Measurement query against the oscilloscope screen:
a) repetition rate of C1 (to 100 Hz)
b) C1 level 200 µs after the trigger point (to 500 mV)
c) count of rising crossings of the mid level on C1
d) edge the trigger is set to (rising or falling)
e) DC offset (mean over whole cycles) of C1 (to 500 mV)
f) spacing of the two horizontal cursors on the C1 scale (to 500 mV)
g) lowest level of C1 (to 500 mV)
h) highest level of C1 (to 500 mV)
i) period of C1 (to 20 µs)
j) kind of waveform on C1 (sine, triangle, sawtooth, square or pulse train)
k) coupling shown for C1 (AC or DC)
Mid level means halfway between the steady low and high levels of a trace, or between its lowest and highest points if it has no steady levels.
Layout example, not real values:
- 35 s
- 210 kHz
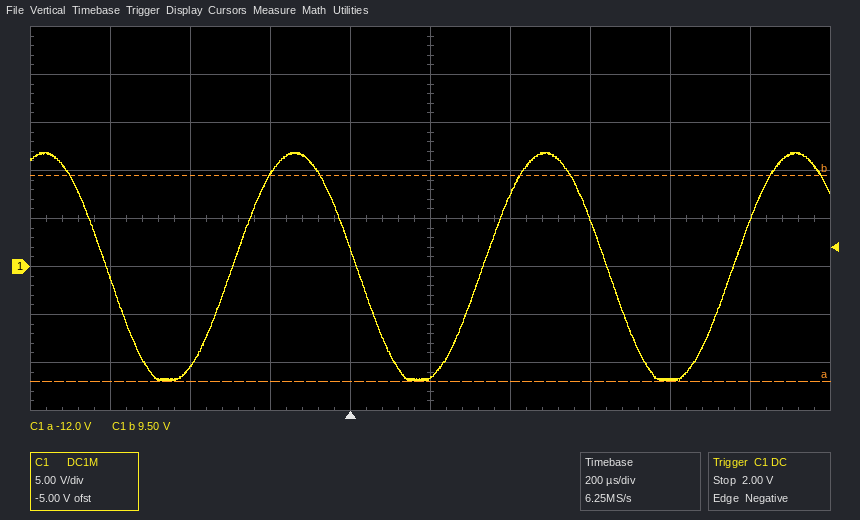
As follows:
- 1.6 kHz
- -11.5 V
- 3
- falling
- 0.0 V
- 21.5 V
- -12.0 V
- 12.0 V
- 620 µs
- sine
- DC
